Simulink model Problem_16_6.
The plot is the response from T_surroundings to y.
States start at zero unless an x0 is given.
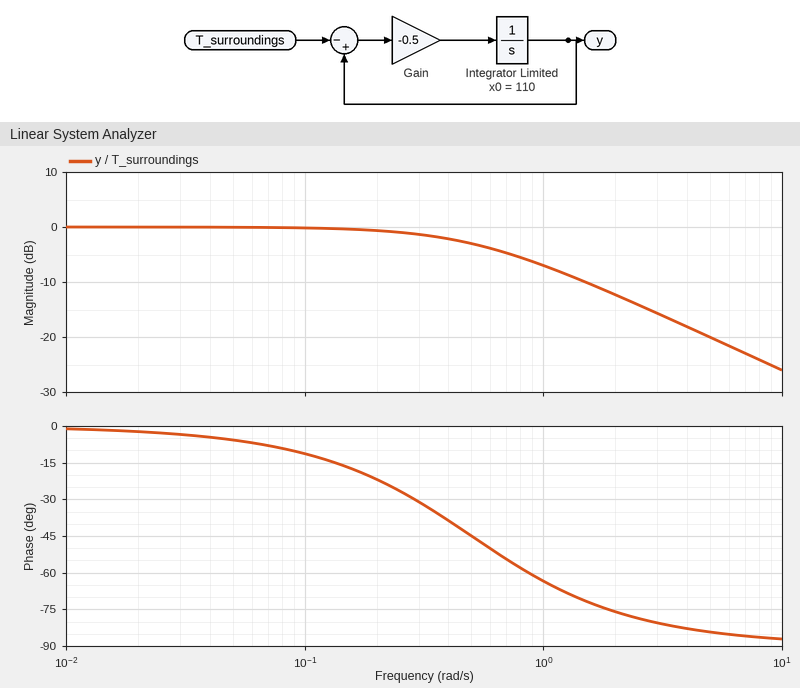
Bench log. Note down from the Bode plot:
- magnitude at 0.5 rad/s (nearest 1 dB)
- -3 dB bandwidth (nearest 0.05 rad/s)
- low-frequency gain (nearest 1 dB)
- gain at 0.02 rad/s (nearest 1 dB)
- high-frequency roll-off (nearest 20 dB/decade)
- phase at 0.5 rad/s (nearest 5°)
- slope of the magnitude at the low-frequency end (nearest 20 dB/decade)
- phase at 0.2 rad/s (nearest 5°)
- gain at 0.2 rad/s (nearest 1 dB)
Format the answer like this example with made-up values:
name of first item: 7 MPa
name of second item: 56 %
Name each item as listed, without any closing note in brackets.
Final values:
magnitude at 0.5 rad/s: -3 dB
-3 dB bandwidth: 0.50 rad/s
low-frequency gain: 0 dB
gain at 0.02 rad/s: 0 dB
high-frequency roll-off: -20 dB/decade
phase at 0.5 rad/s: -45°
slope of the magnitude at the low-frequency end: 0 dB/decade
phase at 0.2 rad/s: -20°
gain at 0.2 rad/s: -1 dB
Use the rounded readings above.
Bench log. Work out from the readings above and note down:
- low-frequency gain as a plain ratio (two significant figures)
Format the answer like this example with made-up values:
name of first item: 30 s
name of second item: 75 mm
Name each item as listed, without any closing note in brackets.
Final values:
low-frequency gain as a plain ratio: 1.0
